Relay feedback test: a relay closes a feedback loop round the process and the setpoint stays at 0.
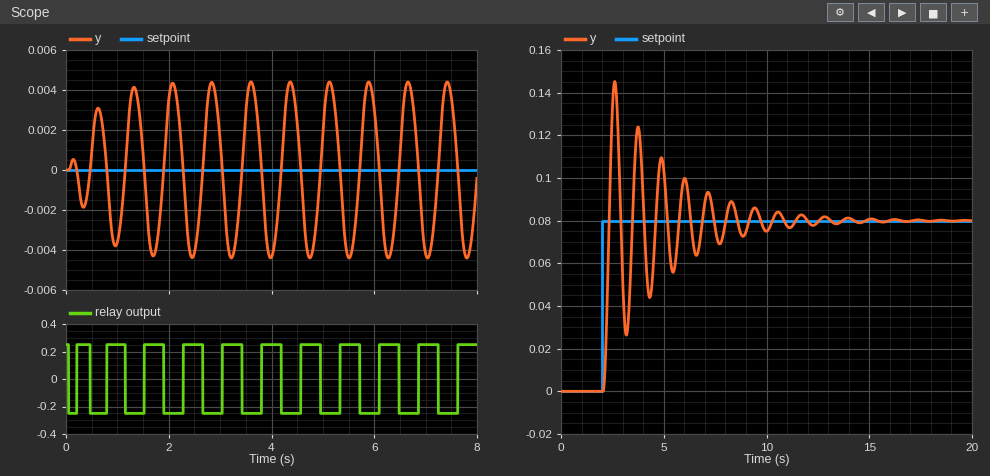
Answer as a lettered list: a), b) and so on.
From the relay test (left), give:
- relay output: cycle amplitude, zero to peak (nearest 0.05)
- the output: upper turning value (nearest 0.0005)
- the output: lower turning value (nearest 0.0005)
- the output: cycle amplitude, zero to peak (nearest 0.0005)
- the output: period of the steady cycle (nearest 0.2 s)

a) 0.25
b) 0.0045
c) -0.0045
d) 0.0045
e) 0.8 s
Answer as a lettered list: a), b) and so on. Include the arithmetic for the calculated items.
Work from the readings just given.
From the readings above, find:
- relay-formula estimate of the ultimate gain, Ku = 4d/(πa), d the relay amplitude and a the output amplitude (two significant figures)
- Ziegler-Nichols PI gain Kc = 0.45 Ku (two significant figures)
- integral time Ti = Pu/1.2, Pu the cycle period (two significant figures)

a) 4 × 0.25 / (π × 0.0045) = 71
b) 0.45 × 71 = 32
c) 0.8 / 1.2 = 0.67 s
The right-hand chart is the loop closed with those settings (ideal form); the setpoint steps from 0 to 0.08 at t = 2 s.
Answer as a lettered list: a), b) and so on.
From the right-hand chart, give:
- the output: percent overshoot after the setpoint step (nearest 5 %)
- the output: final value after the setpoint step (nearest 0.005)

a) 80 %
b) 0.080
